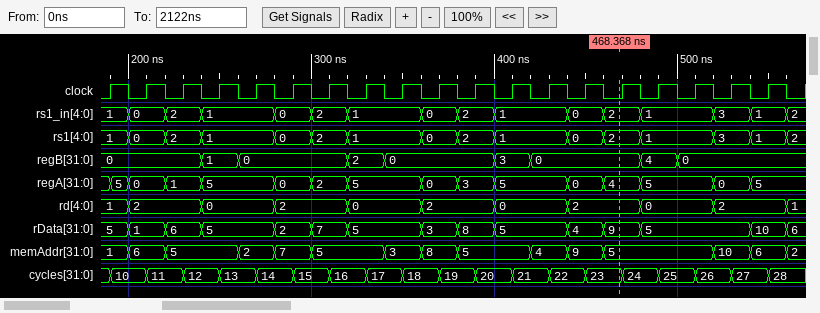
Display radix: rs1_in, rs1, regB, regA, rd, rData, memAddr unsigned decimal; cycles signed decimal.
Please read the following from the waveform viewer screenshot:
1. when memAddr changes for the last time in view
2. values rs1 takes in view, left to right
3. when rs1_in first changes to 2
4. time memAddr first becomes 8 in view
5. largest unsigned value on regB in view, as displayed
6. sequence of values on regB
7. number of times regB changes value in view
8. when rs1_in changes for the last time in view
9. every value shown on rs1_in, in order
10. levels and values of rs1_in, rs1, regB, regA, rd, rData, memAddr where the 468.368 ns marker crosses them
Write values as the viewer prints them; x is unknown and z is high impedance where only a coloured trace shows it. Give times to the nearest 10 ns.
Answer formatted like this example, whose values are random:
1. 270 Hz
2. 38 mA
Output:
1. 560 ns
2. 1, 0, 2, 1, 0, 2, 1, 0, 2, 1, 0, 2, 1, 3, 1, 2
3. 220 ns
4. 360 ns
5. 4
6. 0, 1, 0, 2, 0, 3, 0, 4, 0
7. 8
8. 560 ns
9. 1, 0, 2, 1, 0, 2, 1, 0, 2, 1, 0, 2, 1, 3, 1, 2
10. rs1_in=2, rs1=2, regB=0, regA=4, rd=2, rData=9, memAddr=5
